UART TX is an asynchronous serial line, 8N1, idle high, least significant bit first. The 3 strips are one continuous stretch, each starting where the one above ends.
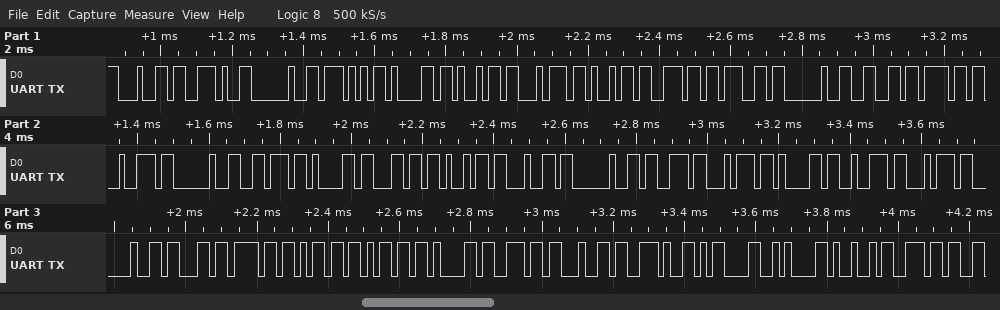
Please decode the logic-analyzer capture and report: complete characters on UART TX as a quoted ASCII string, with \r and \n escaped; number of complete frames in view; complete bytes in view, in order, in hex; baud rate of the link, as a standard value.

"d. Waiting for valid start command.\r\nIn"
39
0x64 0x2E 0x20 0x57 0x61 0x69 0x74 0x69 0x6E 0x67 0x20 0x66 0x6F 0x72 0x20 0x76 0x61 0x6C 0x69 0x64 0x20 0x73 0x74 0x61 0x72 0x74 0x20 0x63 0x6F 0x6D 0x6D 0x61 0x6E 0x64 0x2E 0x0D 0x0A 0x49 0x6E
57600 baud
